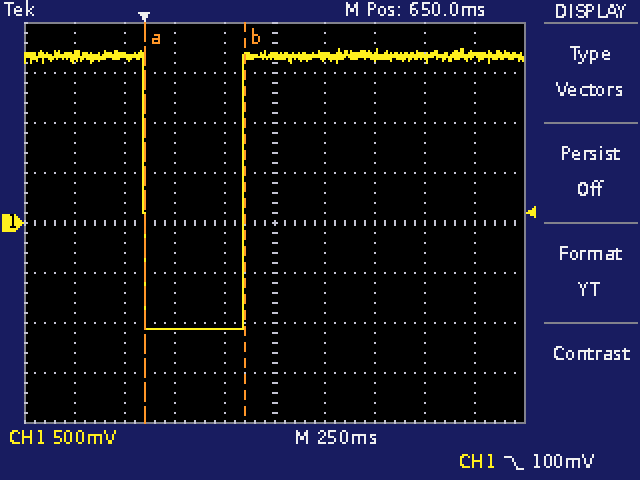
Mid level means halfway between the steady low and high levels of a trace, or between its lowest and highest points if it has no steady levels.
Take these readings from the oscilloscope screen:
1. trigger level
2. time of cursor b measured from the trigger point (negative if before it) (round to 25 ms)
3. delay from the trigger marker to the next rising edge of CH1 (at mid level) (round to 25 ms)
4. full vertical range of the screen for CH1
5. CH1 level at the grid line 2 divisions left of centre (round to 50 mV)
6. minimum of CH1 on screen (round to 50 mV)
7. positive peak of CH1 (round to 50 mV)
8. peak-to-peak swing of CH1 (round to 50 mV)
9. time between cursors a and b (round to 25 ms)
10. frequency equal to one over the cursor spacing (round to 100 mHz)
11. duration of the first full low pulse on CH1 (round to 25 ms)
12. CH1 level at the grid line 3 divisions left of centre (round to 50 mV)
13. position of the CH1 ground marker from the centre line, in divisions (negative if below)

100 mV
+500 ms
500 ms
4 V
-1.05 V
-1.05 V
1.75 V
2.80 V
500 ms
2.0 Hz
500 ms
1.65 V
0.0 div
